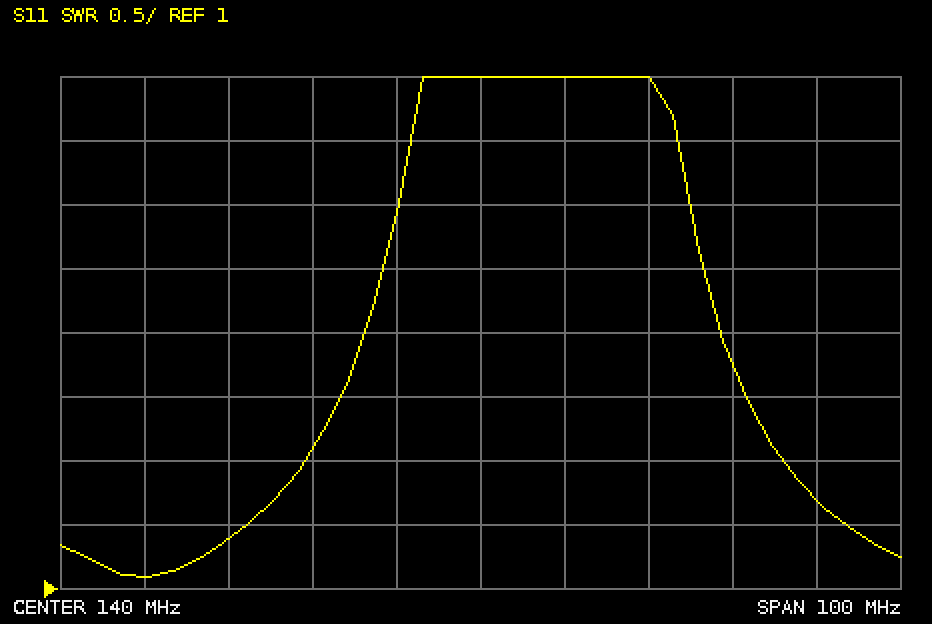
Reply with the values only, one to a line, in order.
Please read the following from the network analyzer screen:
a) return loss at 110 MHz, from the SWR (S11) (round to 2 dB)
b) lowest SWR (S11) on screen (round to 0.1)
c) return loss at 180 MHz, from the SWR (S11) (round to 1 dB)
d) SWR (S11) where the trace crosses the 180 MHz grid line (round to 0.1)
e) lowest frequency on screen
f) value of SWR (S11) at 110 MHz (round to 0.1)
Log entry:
16 dB
1.1
12 dB
1.7
90 MHz
1.4
